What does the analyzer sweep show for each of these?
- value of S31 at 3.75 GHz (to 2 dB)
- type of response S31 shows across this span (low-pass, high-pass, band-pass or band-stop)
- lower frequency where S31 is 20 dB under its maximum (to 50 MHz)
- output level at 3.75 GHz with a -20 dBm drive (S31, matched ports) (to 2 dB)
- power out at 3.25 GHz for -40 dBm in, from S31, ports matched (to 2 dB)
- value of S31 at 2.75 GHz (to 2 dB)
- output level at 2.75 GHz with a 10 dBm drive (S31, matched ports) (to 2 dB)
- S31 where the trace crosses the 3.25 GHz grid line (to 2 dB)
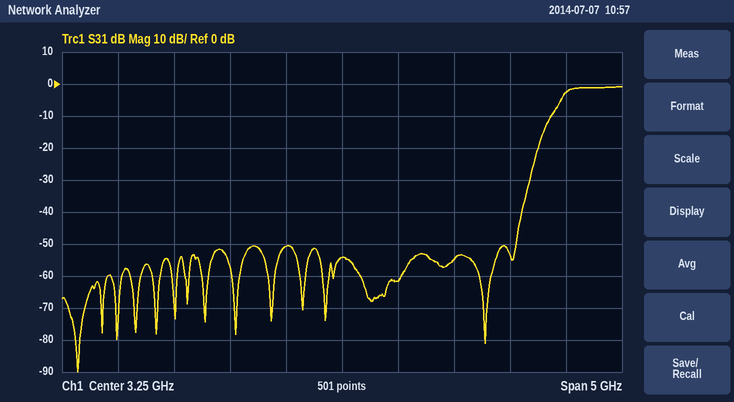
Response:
-62 dB
high-pass
5.00 GHz
-82 dBm
-94 dBm
-50 dB
-40 dBm
-54 dB
